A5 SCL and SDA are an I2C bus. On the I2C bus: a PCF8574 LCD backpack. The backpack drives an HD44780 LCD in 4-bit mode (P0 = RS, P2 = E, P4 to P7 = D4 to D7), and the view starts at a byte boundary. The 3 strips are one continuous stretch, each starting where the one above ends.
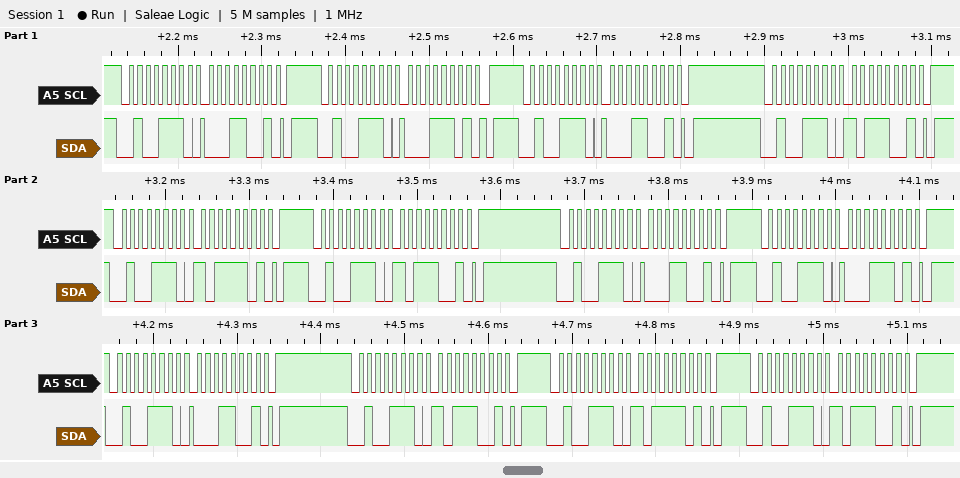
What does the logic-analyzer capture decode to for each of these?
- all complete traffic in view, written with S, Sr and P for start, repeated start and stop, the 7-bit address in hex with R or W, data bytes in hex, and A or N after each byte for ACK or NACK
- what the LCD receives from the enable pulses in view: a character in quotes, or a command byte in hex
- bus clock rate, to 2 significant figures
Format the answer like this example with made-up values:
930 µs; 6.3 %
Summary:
S 27W A 19 A P S 27W A 1D A P S 27W A 19 A P S 27W A B9 A P S 27W A BD A P S 27W A B9 A P S 27W A 19 A P S 27W A 1D A P S 27W A 19 A P S 27W A B9 A P S 27W A BD A P S 27W A B9 A P; data 0x1B data 0x1B; 100 kHz
